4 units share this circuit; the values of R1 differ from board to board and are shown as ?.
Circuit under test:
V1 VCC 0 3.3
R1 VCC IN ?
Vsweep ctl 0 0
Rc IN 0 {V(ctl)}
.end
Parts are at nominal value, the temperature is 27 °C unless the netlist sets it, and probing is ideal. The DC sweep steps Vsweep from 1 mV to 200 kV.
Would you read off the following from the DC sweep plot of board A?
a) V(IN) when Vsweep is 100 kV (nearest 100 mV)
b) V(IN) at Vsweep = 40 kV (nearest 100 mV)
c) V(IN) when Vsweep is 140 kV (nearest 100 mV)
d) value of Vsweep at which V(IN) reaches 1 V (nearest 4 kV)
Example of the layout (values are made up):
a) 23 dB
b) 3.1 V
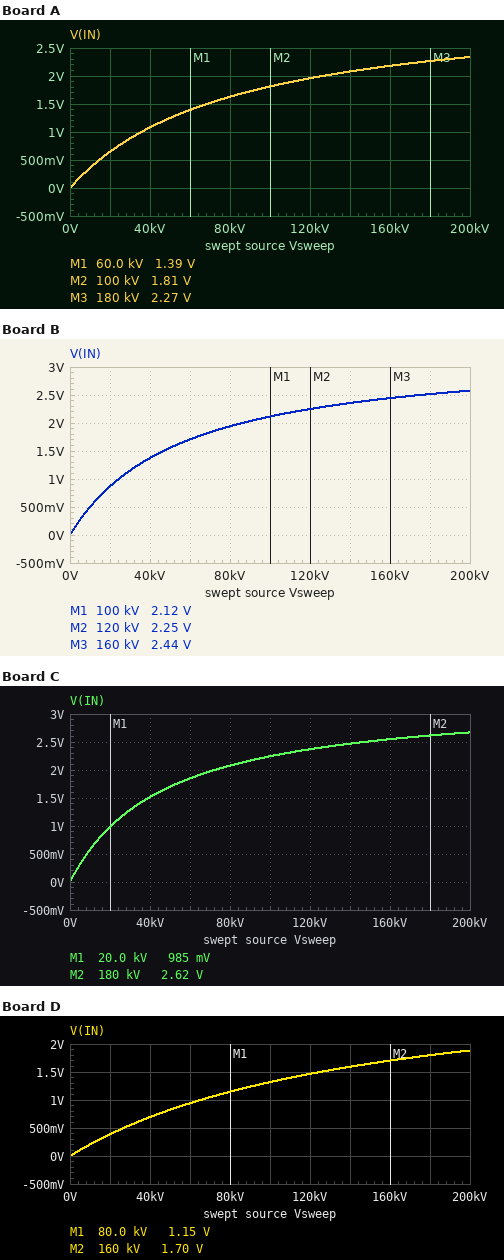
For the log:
a) 1.8 V
b) 1.1 V
c) 2.1 V
d) 36 kV
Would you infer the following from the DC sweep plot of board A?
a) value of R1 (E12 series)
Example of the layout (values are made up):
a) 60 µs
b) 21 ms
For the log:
a) 82 kΩ
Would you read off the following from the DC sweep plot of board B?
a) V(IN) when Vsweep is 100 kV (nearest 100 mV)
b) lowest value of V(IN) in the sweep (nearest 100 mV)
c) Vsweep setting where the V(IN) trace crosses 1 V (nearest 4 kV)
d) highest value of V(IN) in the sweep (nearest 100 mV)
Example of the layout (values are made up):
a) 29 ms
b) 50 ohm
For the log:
a) 2.1 V
b) 0 V
c) 24 kV
d) 2.6 V
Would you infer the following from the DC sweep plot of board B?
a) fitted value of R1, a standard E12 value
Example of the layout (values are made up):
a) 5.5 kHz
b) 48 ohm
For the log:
a) 56 kΩ
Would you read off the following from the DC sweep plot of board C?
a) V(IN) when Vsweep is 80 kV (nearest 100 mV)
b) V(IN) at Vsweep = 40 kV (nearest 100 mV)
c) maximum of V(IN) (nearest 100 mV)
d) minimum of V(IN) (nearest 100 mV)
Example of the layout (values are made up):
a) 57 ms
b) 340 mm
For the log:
a) 2.1 V
b) 1.5 V
c) 2.7 V
d) 0 V
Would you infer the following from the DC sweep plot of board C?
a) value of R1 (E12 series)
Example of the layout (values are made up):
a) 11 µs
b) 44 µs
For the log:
a) 47 kΩ
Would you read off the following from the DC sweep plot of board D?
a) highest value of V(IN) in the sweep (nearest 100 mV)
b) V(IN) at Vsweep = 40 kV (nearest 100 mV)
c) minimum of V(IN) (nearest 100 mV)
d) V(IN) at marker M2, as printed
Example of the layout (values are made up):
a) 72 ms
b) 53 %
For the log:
a) 1.9 V
b) 700 mV
c) 0 V
d) 1.70 V
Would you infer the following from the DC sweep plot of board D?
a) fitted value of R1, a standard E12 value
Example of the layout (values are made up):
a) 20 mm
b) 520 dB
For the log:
a) 150 kΩ
